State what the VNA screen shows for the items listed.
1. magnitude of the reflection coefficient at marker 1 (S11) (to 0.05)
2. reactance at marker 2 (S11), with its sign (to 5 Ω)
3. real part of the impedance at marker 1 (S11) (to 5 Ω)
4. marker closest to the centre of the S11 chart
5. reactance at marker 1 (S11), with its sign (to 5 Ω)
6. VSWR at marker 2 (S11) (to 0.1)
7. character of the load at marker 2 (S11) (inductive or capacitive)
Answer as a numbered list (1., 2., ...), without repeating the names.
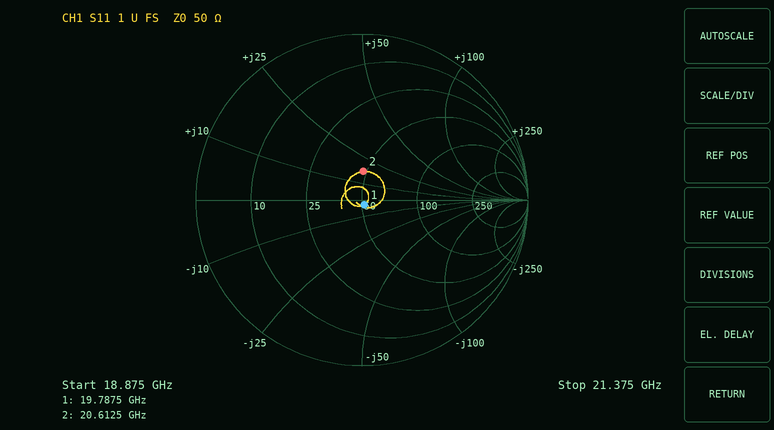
1. 0.05
2. +15 Ω
3. 50 Ω
4. marker 1
5. -5 Ω
6. 1.4
7. inductive
